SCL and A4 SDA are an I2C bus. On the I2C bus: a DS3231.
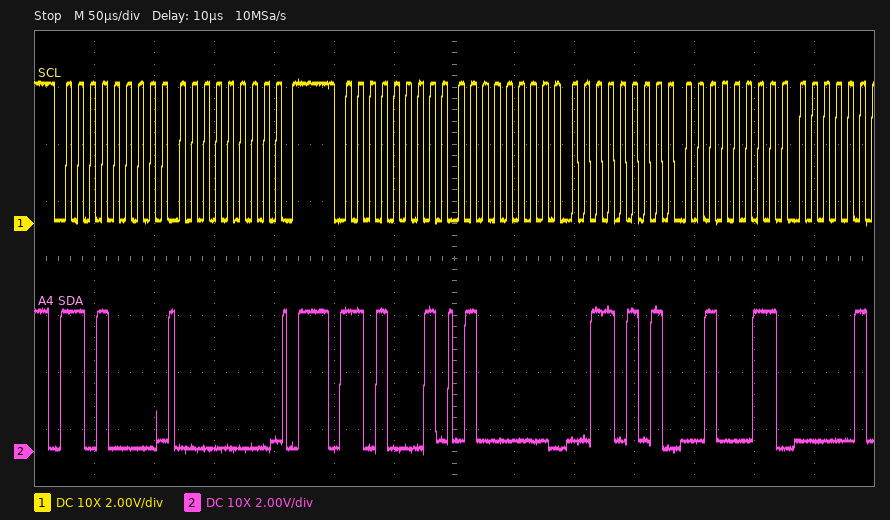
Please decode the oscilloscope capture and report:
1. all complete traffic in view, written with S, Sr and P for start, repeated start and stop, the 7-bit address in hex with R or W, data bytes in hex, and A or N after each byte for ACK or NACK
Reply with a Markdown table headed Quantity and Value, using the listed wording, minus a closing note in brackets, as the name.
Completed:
| Quantity | Value |
|---|---|
| all complete traffic in view, written with S, Sr and P for start, repeated start and stop, the 7-bit address in hex with R or W, data bytes in hex, and A or N after each byte for ACK or NACK | S 68W A 00 A P S 68R A 40 A 35 A 23 A |
